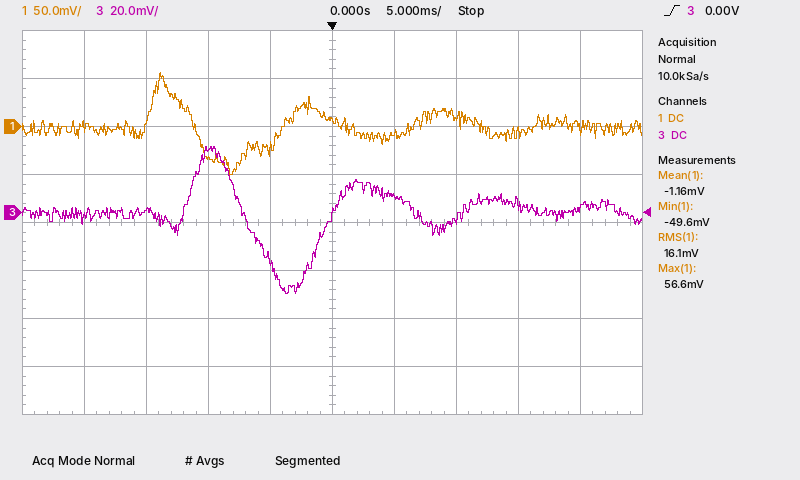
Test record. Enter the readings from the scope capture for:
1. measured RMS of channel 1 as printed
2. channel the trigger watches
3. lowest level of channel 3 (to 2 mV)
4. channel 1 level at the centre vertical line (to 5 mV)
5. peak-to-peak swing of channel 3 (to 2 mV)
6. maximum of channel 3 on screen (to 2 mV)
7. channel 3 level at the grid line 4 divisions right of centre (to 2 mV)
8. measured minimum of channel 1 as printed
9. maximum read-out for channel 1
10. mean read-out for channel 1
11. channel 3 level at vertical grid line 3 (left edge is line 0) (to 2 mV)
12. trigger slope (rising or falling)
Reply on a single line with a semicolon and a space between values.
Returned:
16.1 mV; channel 3; -34 mV; 5 mV; 62 mV; 28 mV; 2 mV; -49.6 mV; 56.6 mV; -1.16 mV; 26 mV; rising
